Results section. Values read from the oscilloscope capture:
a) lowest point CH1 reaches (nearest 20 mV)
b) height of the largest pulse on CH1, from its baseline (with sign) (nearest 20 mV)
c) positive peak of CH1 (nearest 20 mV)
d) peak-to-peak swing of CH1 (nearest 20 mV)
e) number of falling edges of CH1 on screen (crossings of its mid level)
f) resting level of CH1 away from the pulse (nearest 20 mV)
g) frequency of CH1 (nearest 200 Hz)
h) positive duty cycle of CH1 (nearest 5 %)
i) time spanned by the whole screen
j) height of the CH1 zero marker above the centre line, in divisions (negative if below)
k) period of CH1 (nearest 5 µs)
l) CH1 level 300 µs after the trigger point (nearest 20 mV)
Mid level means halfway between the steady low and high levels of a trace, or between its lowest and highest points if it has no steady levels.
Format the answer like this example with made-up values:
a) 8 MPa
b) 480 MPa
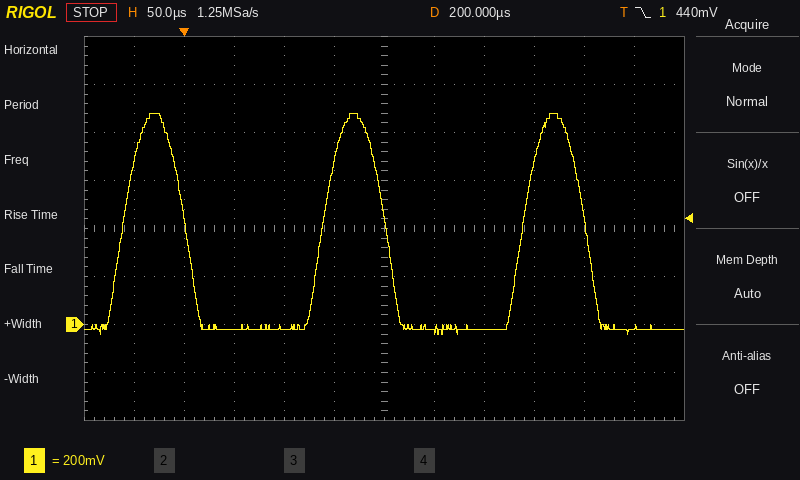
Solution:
a) -40 mV
b) +900 mV
c) 880 mV
d) 920 mV
e) 3
f) -20 mV
g) 5.0 kHz
h) 30 %
i) 600 µs
j) -2.0 div
k) 200 µs
l) -20 mV
